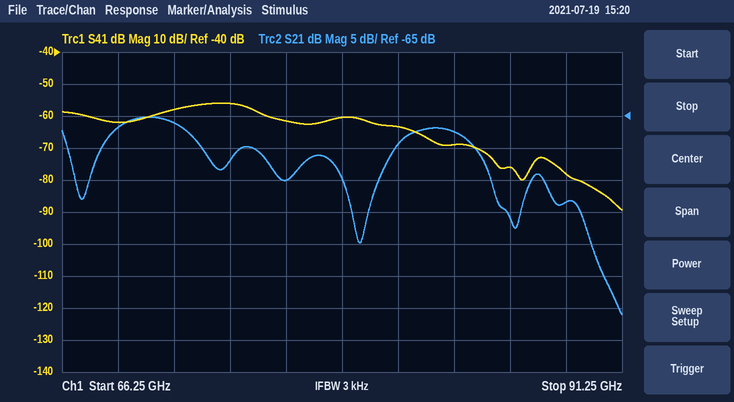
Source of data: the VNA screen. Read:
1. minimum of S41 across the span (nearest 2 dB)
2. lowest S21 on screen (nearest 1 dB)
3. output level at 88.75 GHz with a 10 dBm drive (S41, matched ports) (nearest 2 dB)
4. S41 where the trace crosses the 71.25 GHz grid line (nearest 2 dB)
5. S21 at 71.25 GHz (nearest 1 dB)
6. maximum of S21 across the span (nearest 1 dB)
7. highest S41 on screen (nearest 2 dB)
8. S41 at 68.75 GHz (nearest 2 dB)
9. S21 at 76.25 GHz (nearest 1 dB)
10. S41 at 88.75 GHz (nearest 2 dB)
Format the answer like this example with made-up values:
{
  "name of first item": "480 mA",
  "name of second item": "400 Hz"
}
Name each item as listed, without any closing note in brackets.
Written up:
{
  "minimum of S41 across the span": "-90 dB",
  "lowest S21 on screen": "-96 dB",
  "output level at 88.75 GHz with a 10 dBm drive (S41, matched ports)": "-68 dBm",
  "S41 where the trace crosses the 71.25 GHz grid line": "-58 dB",
  "S21 at 71.25 GHz": "-66 dB",
  "maximum of S21 across the span": "-65 dB",
  "highest S41 on screen": "-56 dB",
  "S41 at 68.75 GHz": "-62 dB",
  "S21 at 76.25 GHz": "-75 dB",
  "S41 at 88.75 GHz": "-78 dB"
}
